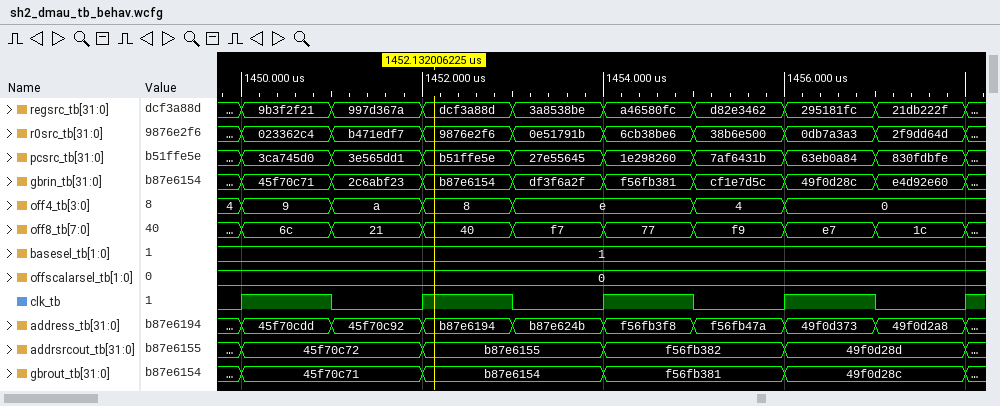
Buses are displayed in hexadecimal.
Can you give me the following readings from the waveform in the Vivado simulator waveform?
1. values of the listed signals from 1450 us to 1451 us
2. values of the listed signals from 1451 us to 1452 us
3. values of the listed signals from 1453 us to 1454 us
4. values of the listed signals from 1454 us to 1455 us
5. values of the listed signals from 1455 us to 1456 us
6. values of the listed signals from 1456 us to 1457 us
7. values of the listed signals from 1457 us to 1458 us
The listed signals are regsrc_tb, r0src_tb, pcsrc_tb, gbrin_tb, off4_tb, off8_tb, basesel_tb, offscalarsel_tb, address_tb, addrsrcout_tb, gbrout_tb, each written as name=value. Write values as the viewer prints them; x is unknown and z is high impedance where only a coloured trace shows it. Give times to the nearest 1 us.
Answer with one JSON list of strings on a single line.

["regsrc_tb=9b3f2f21, r0src_tb=023362c4, pcsrc_tb=3ca745d0, gbrin_tb=45f70c71, off4_tb=9, off8_tb=6c, basesel_tb=1, offscalarsel_tb=0, address_tb=45f70cdd, addrsrcout_tb=45f70c72, gbrout_tb=45f70c71", "regsrc_tb=997d367a, r0src_tb=b471edf7, pcsrc_tb=3e565dd1, gbrin_tb=2c6abf23, off4_tb=a, off8_tb=21, basesel_tb=1, offscalarsel_tb=0, address_tb=45f70c92, addrsrcout_tb=45f70c72, gbrout_tb=45f70c71", "regsrc_tb=3a8538be, r0src_tb=0e51791b, pcsrc_tb=27e55645, gbrin_tb=df3f6a2f, off4_tb=e, off8_tb=f7, basesel_tb=1, offscalarsel_tb=0, address_tb=b87e624b, addrsrcout_tb=b87e6155, gbrout_tb=b87e6154", "regsrc_tb=a46580fc, r0src_tb=6cb38be6, pcsrc_tb=1e298260, gbrin_tb=f56fb381, off4_tb=e, off8_tb=77, basesel_tb=1, offscalarsel_tb=0, address_tb=f56fb3f8, addrsrcout_tb=f56fb382, gbrout_tb=f56fb381", "regsrc_tb=d82e3462, r0src_tb=38b6e500, pcsrc_tb=7af6431b, gbrin_tb=cf1e7d5c, off4_tb=4, off8_tb=f9, basesel_tb=1, offscalarsel_tb=0, address_tb=f56fb47a, addrsrcout_tb=f56fb382, gbrout_tb=f56fb381", "regsrc_tb=295181fc, r0src_tb=0db7a3a3, pcsrc_tb=63eb0a84, gbrin_tb=49f0d28c, off4_tb=0, off8_tb=e7, basesel_tb=1, offscalarsel_tb=0, address_tb=49f0d373, addrsrcout_tb=49f0d28d, gbrout_tb=49f0d28c", "regsrc_tb=21db222f, r0src_tb=2f9dd64d, pcsrc_tb=830fdbfe, gbrin_tb=e4d92e60, off4_tb=0, off8_tb=1c, basesel_tb=1, offscalarsel_tb=0, address_tb=49f0d2a8, addrsrcout_tb=49f0d28d, gbrout_tb=49f0d28c"]
